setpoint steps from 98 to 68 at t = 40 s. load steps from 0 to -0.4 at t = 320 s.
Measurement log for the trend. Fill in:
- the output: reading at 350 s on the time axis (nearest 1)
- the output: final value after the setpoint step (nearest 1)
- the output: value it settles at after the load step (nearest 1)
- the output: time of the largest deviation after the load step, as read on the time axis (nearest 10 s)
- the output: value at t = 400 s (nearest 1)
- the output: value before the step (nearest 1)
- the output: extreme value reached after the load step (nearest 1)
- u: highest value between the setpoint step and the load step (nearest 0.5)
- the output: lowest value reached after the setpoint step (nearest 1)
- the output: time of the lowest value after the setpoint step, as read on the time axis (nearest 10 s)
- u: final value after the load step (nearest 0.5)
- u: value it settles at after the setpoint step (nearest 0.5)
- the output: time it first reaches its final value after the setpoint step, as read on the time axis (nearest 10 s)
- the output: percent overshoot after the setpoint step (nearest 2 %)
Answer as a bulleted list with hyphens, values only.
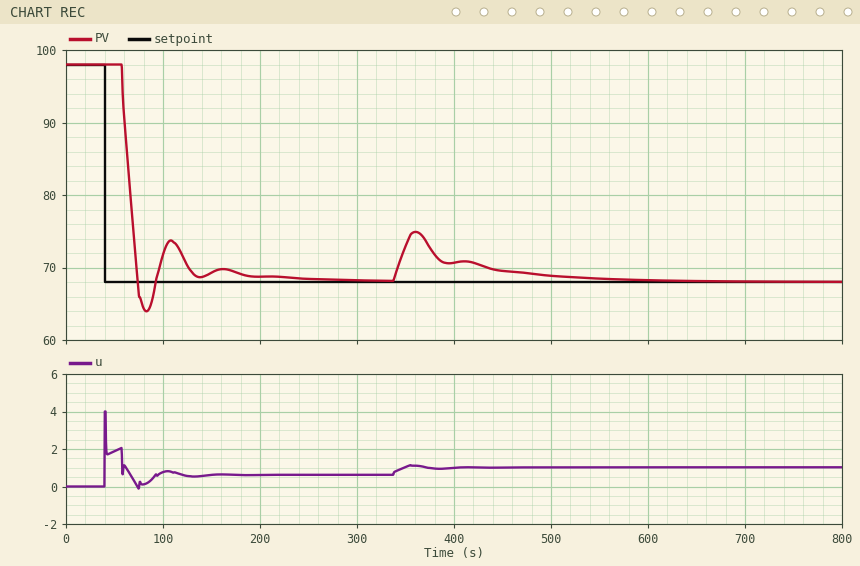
- 73
- 68
- 68
- 360 s
- 71
- 98
- 75
- 4.0
- 64
- 80 s
- 1.0
- 0.5
- 70 s
- 14 %
